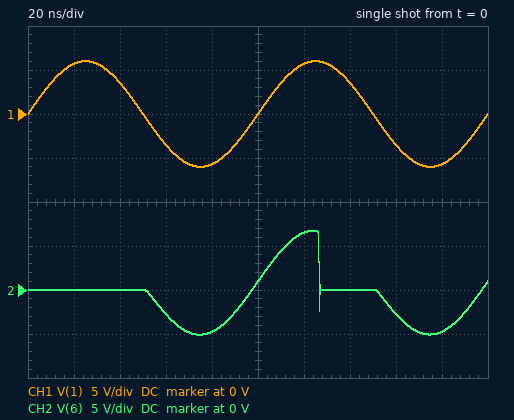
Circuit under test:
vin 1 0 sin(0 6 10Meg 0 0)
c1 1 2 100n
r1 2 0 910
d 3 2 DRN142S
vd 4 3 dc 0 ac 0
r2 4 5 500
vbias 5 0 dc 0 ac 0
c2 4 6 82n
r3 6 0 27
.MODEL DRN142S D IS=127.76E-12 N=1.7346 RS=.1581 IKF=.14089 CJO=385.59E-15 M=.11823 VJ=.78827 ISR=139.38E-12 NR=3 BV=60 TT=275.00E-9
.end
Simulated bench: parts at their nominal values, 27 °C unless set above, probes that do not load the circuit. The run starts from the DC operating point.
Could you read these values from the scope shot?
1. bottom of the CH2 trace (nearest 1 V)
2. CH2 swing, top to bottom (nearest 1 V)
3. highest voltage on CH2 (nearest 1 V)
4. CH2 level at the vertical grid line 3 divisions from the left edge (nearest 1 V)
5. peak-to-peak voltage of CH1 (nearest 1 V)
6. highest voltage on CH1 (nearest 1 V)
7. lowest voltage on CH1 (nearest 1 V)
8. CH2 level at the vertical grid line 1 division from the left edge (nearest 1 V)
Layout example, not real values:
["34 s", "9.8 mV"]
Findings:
["-5 V", "12 V", "7 V", "-3 V", "12 V", "6 V", "-6 V", "0 V"]
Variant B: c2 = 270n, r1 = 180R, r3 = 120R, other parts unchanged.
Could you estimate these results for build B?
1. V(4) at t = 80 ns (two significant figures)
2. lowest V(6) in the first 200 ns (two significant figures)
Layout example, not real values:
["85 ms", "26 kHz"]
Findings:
["-4.9 V", "-5.2 V"]
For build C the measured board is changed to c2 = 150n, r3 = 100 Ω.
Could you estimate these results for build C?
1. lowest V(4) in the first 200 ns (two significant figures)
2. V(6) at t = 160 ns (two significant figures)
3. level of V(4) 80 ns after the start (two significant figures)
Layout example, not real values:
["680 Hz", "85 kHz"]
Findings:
["-5.2 V", "-2.8 V", "-4.9 V"]
